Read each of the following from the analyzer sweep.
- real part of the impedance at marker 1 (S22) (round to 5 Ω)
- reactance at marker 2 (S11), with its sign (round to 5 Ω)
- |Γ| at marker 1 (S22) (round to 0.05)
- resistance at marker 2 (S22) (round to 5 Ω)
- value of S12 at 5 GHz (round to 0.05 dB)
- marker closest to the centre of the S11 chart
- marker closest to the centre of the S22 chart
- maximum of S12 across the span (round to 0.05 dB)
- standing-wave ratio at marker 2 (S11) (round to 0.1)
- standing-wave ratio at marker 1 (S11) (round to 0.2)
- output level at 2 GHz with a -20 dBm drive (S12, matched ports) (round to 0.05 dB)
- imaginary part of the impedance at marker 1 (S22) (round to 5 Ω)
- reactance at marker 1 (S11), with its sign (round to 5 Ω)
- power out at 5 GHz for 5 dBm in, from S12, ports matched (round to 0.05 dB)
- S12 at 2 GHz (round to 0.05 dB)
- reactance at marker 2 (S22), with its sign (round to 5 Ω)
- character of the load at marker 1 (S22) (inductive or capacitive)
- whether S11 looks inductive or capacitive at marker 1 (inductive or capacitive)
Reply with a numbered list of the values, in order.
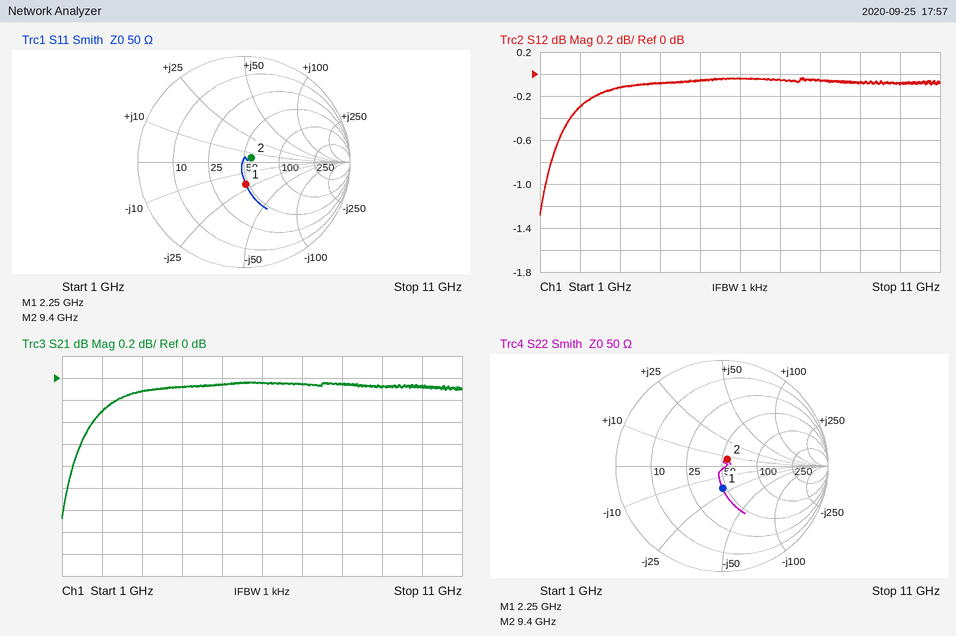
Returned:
1. 45 Ω
2. +5 Ω
3. 0.20
4. 55 Ω
5. -0.05 dB
6. marker 2
7. marker 2
8. -0.05 dB
9. 1.2
10. 1.6
11. -20.30 dBm
12. -20 Ω
13. -20 Ω
14. 4.95 dBm
15. -0.30 dB
16. +5 Ω
17. capacitive
18. capacitive
